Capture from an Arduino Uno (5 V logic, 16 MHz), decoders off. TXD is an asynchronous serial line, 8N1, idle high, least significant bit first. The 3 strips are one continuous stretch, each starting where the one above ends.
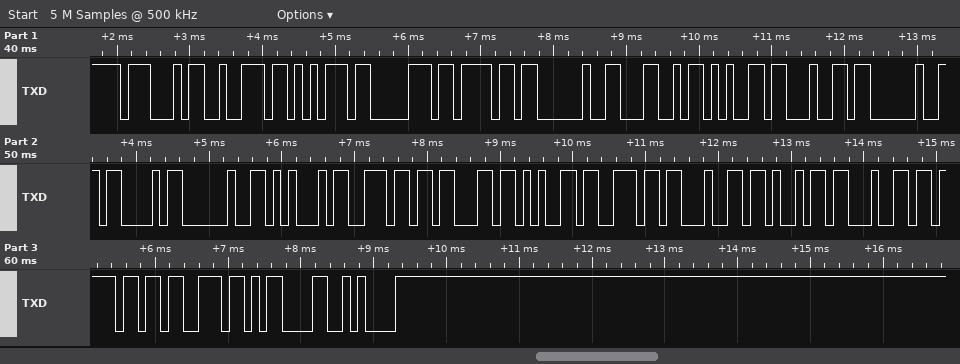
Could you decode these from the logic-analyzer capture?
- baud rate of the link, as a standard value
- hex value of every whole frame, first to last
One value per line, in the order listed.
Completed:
9600 baud
47 72 75 70 6F 20 4C 65 64 20 43 20 45 6E 63 65 6E 64 69 64 6F 73 0D 0A
